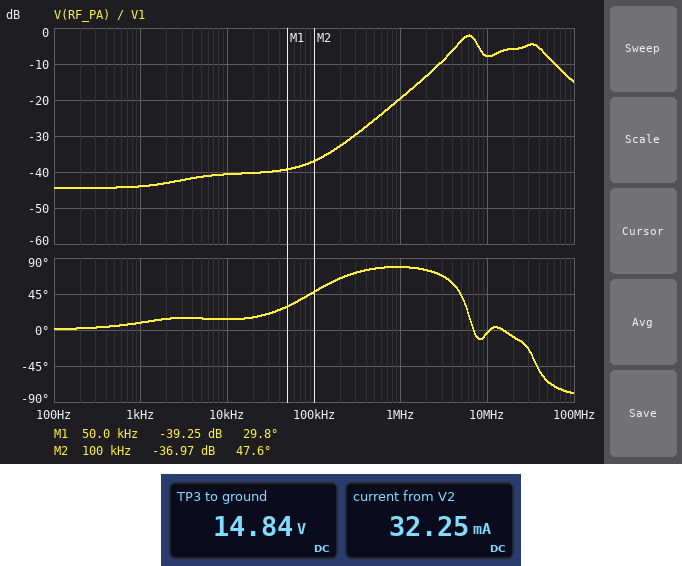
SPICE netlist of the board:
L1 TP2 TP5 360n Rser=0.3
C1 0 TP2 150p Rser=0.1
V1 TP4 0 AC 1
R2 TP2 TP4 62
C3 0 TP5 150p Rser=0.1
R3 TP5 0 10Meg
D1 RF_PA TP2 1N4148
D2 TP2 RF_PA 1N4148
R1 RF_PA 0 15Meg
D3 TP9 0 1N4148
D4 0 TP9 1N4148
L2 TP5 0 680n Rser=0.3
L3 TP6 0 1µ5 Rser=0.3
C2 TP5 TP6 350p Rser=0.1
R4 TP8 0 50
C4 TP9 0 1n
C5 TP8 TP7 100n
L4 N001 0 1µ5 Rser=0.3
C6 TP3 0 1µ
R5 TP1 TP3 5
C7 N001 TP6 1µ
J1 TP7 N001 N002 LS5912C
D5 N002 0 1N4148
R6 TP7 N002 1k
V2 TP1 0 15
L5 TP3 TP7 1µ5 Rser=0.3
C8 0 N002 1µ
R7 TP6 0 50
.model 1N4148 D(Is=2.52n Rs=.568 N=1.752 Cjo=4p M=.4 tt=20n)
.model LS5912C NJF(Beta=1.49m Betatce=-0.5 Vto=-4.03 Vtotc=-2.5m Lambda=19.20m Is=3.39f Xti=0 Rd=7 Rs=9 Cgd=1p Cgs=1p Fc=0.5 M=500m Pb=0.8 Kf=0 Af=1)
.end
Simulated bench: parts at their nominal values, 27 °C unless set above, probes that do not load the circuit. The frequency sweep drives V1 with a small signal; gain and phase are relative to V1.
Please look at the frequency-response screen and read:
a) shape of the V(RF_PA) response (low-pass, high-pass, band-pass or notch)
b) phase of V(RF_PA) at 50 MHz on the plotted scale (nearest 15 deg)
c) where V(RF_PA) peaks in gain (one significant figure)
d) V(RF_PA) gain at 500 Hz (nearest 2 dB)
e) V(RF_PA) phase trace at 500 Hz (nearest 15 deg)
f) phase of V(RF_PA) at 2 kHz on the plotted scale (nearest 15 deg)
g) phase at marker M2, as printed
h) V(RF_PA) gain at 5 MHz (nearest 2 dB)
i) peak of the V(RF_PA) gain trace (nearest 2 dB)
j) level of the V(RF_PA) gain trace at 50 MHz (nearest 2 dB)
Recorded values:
band-pass
-60 deg
6 MHz
-44 dB
0 deg
15 deg
47.6 deg
-4 dB
-2 dB
-8 dB
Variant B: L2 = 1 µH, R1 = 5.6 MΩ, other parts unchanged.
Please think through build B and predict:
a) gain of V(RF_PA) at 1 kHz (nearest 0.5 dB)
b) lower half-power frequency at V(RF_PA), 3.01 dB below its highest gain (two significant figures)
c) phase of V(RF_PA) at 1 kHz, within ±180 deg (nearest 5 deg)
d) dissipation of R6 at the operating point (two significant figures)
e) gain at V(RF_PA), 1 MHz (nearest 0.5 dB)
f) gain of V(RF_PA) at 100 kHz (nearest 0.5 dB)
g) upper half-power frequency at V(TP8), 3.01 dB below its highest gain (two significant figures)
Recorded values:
-48.0 dB
3.7 MHz
15 deg
200 mW
-17.0 dB
-35.5 dB
34 MHz
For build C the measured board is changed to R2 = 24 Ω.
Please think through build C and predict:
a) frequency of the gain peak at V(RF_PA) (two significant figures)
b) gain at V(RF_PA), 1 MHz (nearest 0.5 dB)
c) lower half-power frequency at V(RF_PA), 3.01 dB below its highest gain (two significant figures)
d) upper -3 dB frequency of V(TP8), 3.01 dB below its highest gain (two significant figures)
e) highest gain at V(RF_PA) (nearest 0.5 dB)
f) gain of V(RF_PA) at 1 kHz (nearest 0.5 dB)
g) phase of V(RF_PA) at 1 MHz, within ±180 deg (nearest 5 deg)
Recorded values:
5.8 MHz
-11.5 dB
2.8 MHz
34 MHz
-0.5 dB
-36.0 dB
70 deg
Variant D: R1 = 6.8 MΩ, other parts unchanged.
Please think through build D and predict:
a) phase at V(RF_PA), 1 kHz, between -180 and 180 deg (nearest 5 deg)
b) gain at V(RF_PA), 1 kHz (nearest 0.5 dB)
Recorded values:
15 deg
-47.0 dB
